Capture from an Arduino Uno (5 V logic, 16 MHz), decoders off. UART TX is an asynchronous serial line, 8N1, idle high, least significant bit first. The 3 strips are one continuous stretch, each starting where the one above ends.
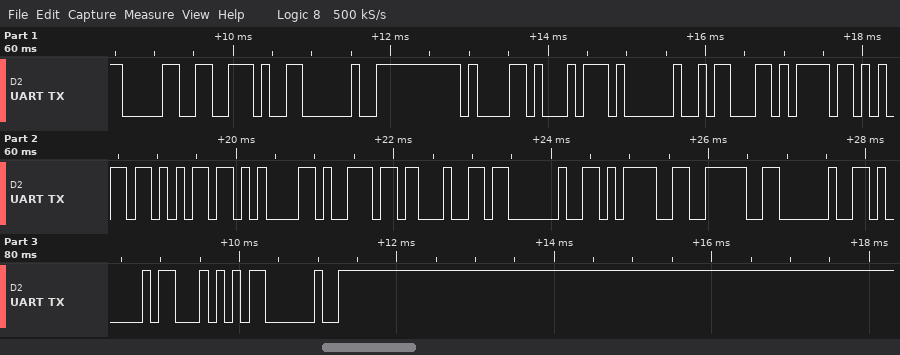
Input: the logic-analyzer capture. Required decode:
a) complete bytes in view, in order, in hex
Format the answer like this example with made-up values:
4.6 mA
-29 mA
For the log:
0x30 0x2E 0x20 0x61 0x74 0x20 0x63 0x6F 0x6D 0x6D 0x61 0x6E 0x64 0x20 0x3D 0x3E 0x20 0x41 0x54 0x20
